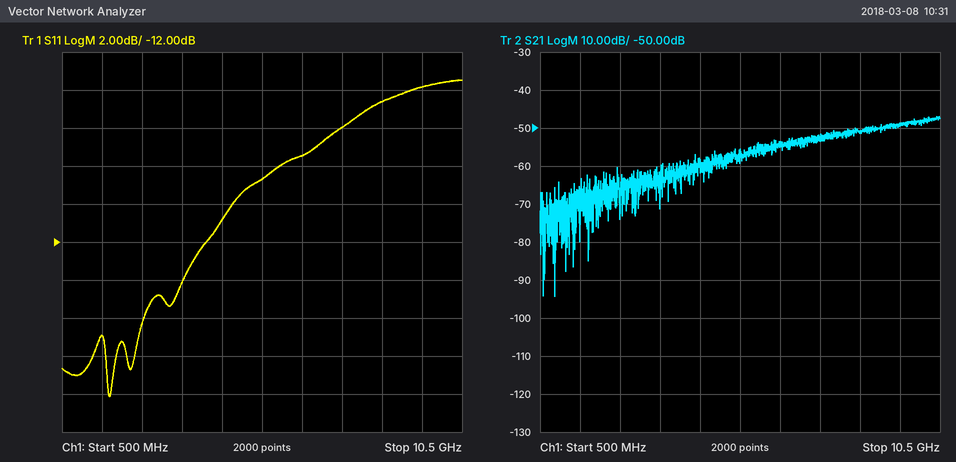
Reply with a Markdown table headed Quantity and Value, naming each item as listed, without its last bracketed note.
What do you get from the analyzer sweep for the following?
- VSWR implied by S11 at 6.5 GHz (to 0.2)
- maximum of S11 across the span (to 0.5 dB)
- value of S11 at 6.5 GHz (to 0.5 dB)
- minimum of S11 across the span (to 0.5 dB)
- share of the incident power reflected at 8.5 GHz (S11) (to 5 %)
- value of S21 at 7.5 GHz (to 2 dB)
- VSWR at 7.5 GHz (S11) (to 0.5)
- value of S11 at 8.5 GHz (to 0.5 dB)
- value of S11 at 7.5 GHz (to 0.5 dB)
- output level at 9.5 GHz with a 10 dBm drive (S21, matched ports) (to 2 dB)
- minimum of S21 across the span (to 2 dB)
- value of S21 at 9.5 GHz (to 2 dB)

| Quantity | Value |
|---|---|
| VSWR implied by S11 at 6.5 GHz | 2.4 |
| maximum of S11 across the span | -3.5 dB |
| value of S11 at 6.5 GHz | -7.5 dB |
| minimum of S11 across the span | -20.0 dB |
| share of the incident power reflected at 8.5 GHz (S11) | 35 % |
| value of S21 at 7.5 GHz | -52 dB |
| VSWR at 7.5 GHz (S11) | 3.0 |
| value of S11 at 8.5 GHz | -4.5 dB |
| value of S11 at 7.5 GHz | -6.0 dB |
| output level at 9.5 GHz with a 10 dBm drive (S21, matched ports) | -40 dBm |
| minimum of S21 across the span | -94 dB |
| value of S21 at 9.5 GHz | -50 dB |
